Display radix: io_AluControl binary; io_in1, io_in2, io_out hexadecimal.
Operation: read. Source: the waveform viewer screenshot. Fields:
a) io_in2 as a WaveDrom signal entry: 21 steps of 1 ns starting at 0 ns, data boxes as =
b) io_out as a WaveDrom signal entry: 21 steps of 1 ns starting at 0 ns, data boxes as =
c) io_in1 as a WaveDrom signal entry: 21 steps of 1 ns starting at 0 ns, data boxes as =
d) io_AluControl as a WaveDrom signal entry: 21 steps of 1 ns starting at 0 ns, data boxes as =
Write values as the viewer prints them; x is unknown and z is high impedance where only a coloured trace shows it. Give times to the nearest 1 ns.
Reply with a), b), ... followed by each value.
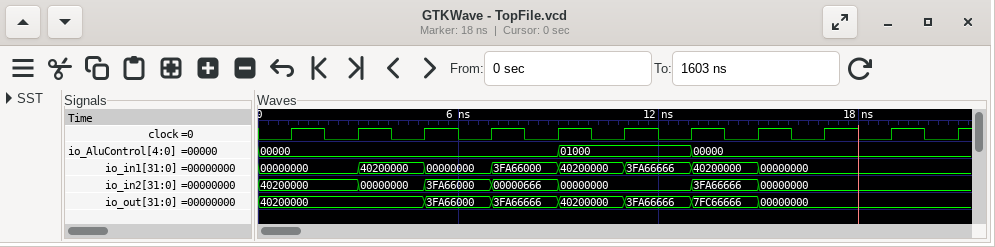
a) {name: 'io_in2', wave: '=..=.=.=.=...=.=.....', data: '40200000 00000000 3FA66000 00000666 00000000 3FA66666 00000000'}
b) {name: 'io_out', wave: '=....=.=.=.=.=.=.....', data: '40200000 3FA66000 3FA66666 40200000 3FA66666 7FC66666 00000000'}
c) {name: 'io_in1', wave: '=..=.=.=.=.=.=.=.....', data: '00000000 40200000 00000000 3FA66000 40200000 3FA66666 40200000 00000000'}
d) {name: 'io_AluControl', wave: '=........=...=.......', data: '00000 01000 00000'}
